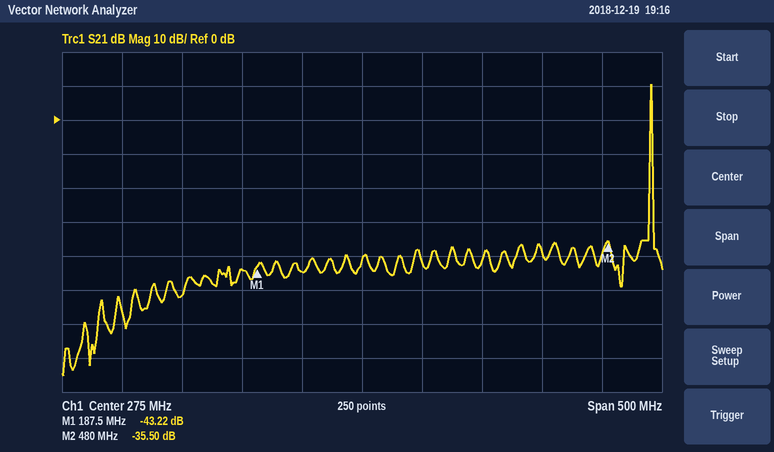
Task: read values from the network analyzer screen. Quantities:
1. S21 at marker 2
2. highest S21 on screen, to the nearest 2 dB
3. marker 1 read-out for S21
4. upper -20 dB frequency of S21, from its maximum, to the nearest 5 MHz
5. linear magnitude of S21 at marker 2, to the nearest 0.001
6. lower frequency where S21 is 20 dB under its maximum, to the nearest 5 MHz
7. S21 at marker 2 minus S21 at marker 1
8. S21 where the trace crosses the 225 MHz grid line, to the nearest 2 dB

-35.50 dB
10 dB
-43.22 dB
515 MHz
0.017
515 MHz
7.72 dB
-44 dB
